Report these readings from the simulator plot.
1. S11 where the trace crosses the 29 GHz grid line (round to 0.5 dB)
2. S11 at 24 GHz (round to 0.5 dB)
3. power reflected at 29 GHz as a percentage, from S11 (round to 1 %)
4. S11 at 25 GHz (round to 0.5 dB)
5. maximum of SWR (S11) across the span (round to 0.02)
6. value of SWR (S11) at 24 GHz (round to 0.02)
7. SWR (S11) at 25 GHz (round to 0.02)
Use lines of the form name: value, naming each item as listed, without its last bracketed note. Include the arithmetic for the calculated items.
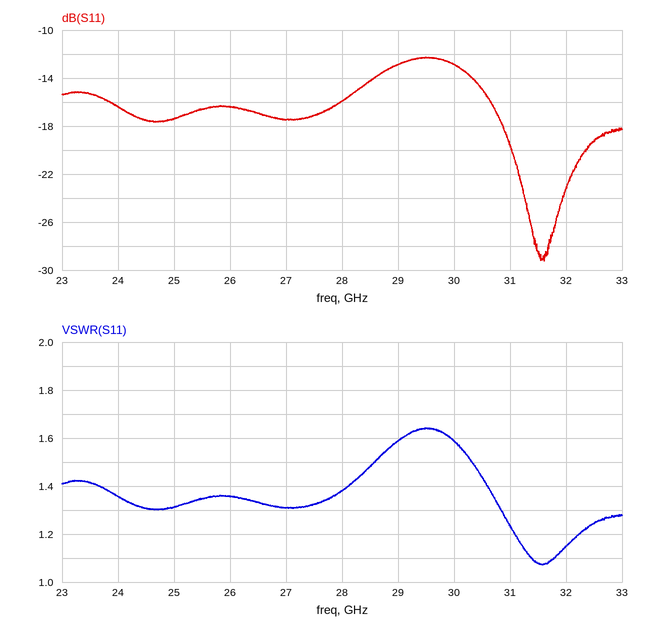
S11 where the trace crosses the 29 GHz grid line: -13.0 dB
S11 at 24 GHz: -16.5 dB
power reflected at 29 GHz as a percentage, from S11: 10^(-13/10) ≈ 5 %
S11 at 25 GHz: -17.5 dB
maximum of SWR (S11) across the span: 1.64
value of SWR (S11) at 24 GHz: 1.36
SWR (S11) at 25 GHz: 1.32
